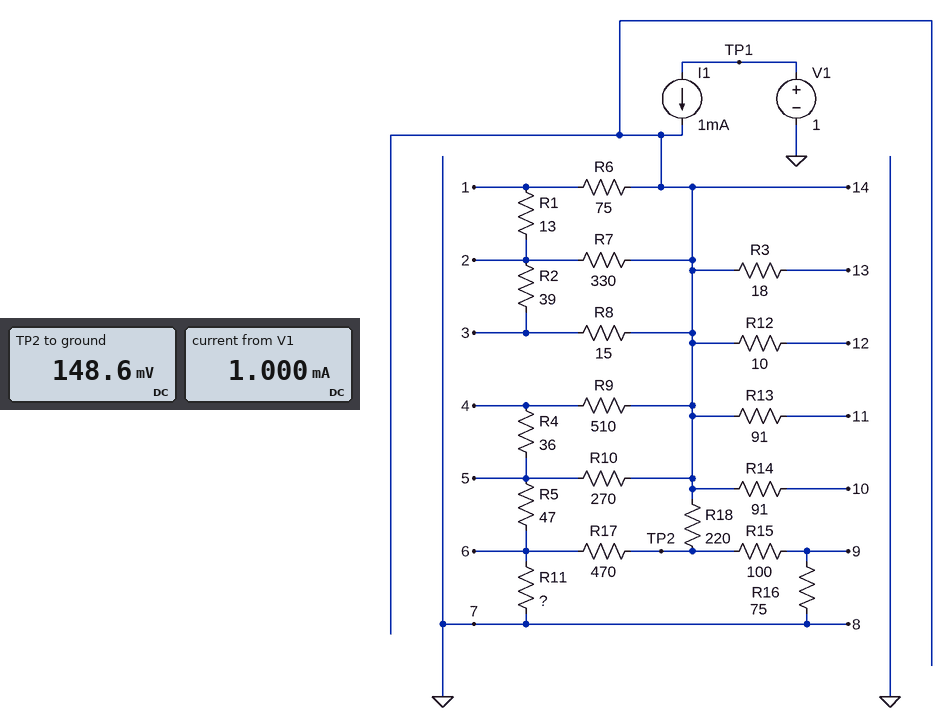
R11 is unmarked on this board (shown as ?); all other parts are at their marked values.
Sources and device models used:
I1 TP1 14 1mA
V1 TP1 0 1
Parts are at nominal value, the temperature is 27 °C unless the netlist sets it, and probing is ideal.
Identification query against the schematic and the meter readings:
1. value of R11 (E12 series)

1.5 kΩ
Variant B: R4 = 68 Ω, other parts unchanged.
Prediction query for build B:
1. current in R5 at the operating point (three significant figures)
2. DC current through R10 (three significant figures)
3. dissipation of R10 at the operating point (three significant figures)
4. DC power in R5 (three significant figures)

316 µA
215 µA
12.5 µW
4.69 µW
